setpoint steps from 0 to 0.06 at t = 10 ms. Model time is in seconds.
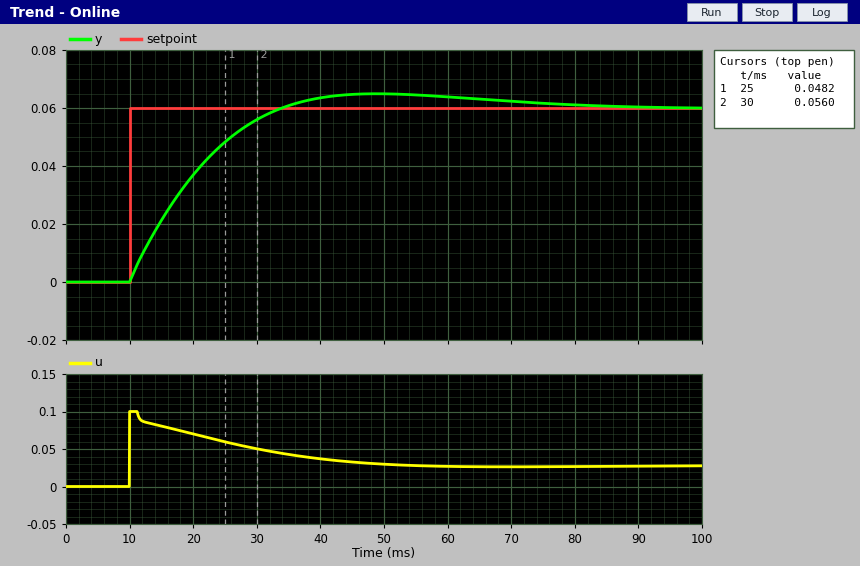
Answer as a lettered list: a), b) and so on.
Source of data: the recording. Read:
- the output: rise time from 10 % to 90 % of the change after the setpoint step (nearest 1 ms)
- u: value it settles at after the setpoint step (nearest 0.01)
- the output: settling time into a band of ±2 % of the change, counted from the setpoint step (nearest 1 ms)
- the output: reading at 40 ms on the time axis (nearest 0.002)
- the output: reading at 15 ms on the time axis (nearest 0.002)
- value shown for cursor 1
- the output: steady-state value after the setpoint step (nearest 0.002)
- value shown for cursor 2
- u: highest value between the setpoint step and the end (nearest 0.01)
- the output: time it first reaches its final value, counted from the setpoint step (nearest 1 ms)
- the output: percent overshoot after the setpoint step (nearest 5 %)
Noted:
a) 17 ms
b) 0.03
c) 69 ms
d) 0.064
e) 0.022
f) 0.0482
g) 0.060
h) 0.0560
i) 0.10
j) 24 ms
k) 10 %
